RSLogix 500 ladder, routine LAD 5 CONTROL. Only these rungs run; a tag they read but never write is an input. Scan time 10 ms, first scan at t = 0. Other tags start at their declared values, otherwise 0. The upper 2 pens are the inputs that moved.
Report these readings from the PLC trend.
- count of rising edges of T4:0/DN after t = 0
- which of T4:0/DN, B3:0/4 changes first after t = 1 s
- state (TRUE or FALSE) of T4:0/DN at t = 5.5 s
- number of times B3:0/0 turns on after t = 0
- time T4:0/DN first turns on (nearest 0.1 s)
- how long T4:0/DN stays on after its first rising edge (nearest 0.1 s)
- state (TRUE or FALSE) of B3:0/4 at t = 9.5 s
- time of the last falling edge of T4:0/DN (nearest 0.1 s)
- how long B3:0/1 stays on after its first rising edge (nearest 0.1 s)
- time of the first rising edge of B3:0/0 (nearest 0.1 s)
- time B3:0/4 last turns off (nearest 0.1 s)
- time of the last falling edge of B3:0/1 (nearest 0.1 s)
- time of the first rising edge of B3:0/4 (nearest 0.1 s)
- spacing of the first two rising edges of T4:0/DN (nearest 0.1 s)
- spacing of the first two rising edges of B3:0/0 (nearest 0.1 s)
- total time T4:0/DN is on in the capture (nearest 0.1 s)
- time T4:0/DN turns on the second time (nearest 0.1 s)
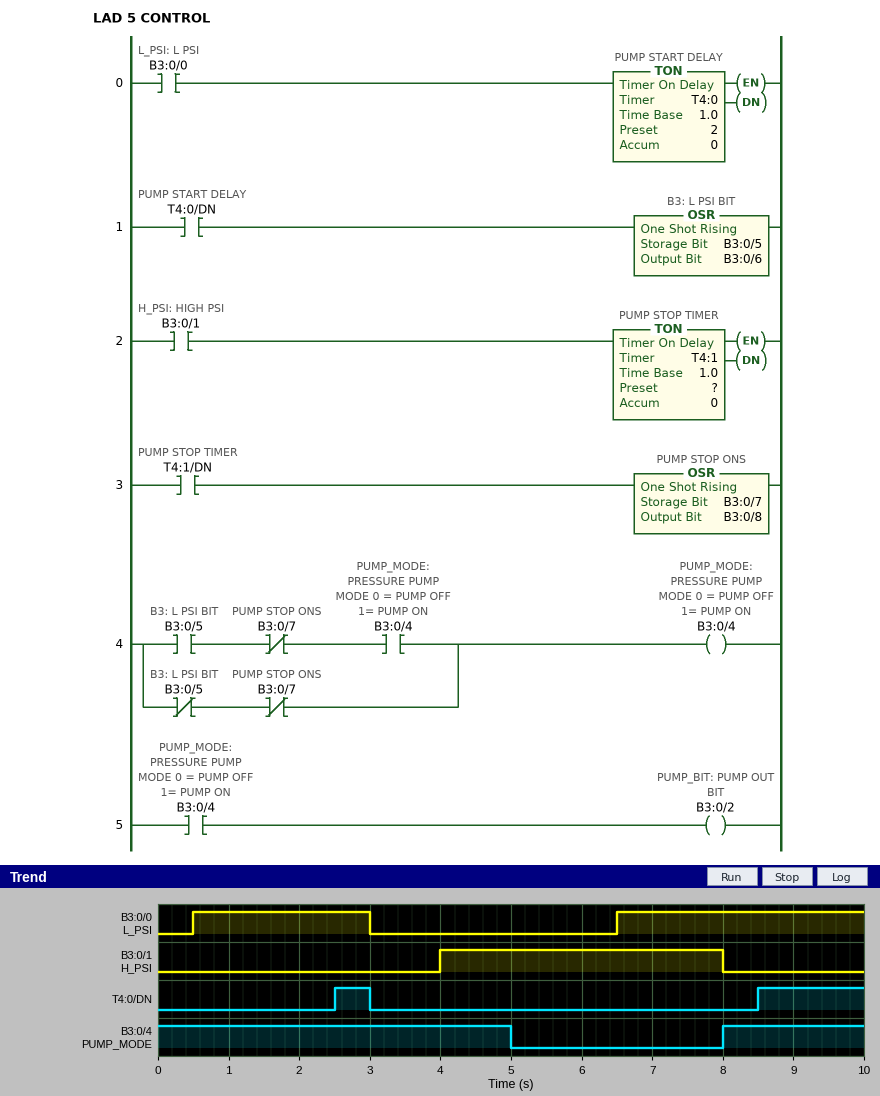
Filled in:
2
T4:0/DN
FALSE
2
2.5 s
0.5 s
TRUE
3.0 s
4.0 s
0.5 s
5.0 s
8.0 s
8.0 s
6.0 s
6.0 s
2.0 s
8.5 s
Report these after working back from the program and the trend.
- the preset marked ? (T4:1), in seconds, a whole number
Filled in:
1 s
